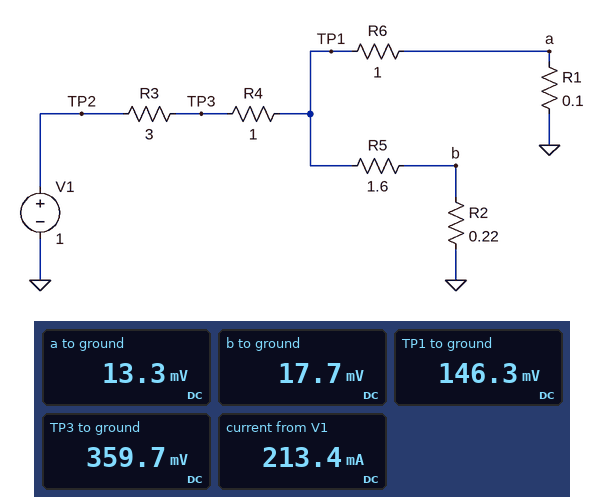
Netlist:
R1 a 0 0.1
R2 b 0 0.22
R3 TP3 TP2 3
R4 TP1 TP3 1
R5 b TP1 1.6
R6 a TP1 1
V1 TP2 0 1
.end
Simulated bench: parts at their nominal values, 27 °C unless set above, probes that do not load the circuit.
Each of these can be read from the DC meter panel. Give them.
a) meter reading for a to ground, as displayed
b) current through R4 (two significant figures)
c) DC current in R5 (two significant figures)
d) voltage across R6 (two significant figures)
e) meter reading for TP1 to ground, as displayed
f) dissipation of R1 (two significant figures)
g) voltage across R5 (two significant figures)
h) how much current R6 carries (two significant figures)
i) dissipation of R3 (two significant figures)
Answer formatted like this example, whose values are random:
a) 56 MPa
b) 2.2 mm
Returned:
a) 13.3 mV
b) 210 mA
c) 80 mA
d) 130 mV
e) 146.3 mV
f) 1.8 mW
g) 130 mV
h) 130 mA
i) 140 mW
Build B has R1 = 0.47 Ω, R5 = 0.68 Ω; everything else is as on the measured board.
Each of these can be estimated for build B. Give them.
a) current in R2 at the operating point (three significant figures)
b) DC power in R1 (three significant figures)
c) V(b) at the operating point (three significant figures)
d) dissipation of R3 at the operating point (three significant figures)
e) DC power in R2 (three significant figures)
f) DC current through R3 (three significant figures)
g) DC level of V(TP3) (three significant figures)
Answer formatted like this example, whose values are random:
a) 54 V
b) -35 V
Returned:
a) 136 mA
b) 3.26 mW
c) 29.9 mV
d) 144 mW
e) 4.07 mW
f) 219 mA
g) 342 mV
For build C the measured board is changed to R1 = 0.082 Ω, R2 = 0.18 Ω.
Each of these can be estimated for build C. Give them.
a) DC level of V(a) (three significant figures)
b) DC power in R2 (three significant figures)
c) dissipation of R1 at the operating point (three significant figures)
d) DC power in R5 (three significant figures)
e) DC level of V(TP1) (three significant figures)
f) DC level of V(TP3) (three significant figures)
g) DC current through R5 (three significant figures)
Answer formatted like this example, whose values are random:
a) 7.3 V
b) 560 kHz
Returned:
a) 10.9 mV
b) 1.18 mW
c) 1.45 mW
d) 10.5 mW
e) 144 mV
f) 358 mV
g) 80.9 mA
